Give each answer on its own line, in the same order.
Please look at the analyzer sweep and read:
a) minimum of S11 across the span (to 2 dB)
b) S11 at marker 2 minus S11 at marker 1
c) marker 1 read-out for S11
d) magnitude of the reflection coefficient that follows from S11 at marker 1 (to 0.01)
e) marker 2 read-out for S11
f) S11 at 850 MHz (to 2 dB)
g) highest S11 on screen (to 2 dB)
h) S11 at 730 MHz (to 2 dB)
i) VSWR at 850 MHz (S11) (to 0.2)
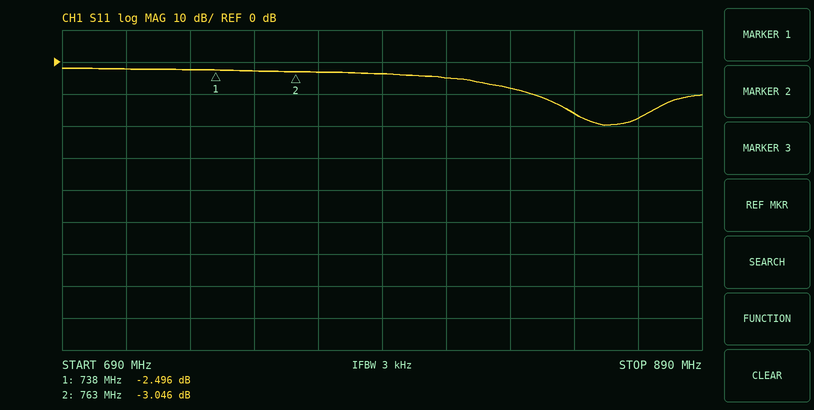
-20 dB
-0.550 dB
-2.496 dB
0.75
-3.046 dB
-16 dB
-2 dB
-2 dB
1.4
